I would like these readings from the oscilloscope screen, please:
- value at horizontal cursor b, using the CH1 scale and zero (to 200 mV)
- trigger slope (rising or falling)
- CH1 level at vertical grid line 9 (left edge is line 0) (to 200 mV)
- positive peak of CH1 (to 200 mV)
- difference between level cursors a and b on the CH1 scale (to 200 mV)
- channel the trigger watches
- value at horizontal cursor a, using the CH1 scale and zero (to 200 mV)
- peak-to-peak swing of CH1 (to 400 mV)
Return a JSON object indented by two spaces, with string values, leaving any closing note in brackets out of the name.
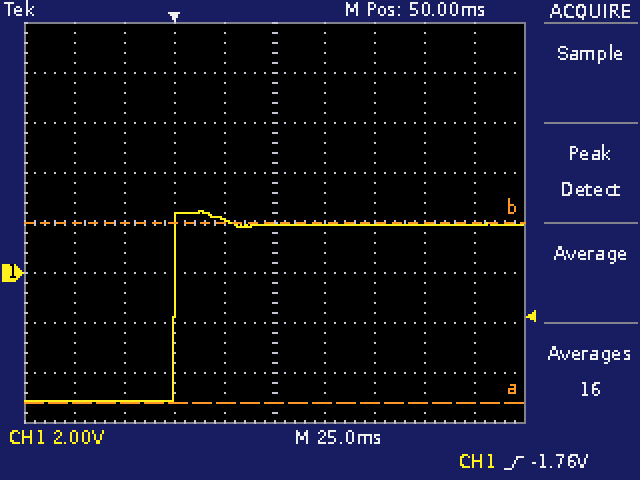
{
  "value at horizontal cursor b, using the CH1 scale and zero": "2.0 V",
  "trigger slope": "rising",
  "CH1 level at vertical grid line 9 (left edge is line 0)": "2.0 V",
  "positive peak of CH1": "2.4 V",
  "difference between level cursors a and b on the CH1 scale": "7.2 V",
  "channel the trigger watches": "CH1",
  "value at horizontal cursor a, using the CH1 scale and zero": "-5.2 V",
  "peak-to-peak swing of CH1": "7.6 V"
}
